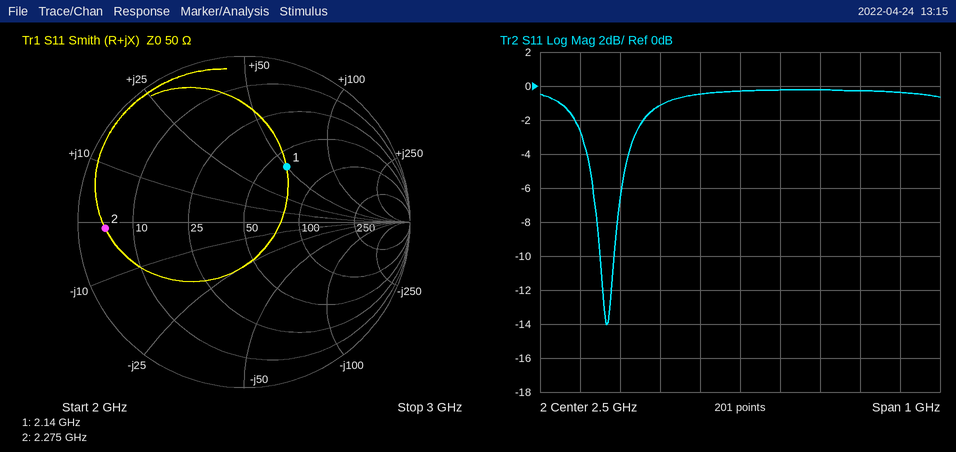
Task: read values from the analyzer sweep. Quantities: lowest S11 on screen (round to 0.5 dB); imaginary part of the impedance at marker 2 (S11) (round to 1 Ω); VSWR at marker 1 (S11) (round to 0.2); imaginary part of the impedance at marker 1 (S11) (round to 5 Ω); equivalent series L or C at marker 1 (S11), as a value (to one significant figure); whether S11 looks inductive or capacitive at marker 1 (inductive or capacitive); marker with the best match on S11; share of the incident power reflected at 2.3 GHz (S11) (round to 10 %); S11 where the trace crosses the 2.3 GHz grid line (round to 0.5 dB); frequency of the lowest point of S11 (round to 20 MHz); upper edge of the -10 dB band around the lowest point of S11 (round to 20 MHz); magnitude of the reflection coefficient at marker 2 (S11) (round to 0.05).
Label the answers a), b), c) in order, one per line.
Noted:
a) -14.0 dB
b) -1 Ω
c) 2.4
d) +50 Ω
e) 4 nH
f) inductive
g) marker 1
h) 80 %
i) -1.0 dB
j) 2.16 GHz
k) 2.18 GHz
l) 0.85
